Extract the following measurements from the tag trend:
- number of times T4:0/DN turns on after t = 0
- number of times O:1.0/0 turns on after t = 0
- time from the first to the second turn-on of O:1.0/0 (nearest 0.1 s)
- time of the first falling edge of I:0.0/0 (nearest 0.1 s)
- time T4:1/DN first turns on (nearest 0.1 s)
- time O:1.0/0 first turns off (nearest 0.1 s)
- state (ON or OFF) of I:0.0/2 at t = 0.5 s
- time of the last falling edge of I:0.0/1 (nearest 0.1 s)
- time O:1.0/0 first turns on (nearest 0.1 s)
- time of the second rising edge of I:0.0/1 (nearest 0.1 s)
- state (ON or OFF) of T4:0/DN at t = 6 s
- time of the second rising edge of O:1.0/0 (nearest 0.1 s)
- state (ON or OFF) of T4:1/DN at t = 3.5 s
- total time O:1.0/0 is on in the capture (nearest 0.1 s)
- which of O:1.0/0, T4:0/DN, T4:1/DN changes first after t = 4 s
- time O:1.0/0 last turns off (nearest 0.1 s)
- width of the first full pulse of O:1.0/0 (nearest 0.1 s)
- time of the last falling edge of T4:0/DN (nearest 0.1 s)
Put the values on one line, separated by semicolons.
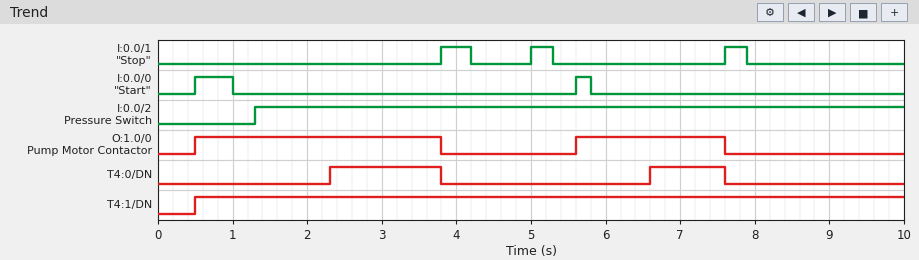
2; 2; 5.1 s; 1.0 s; 0.5 s; 3.8 s; OFF; 7.9 s; 0.5 s; 5.0 s; OFF; 5.6 s; ON; 5.3 s; O:1.0/0; 7.6 s; 3.3 s; 7.6 s
